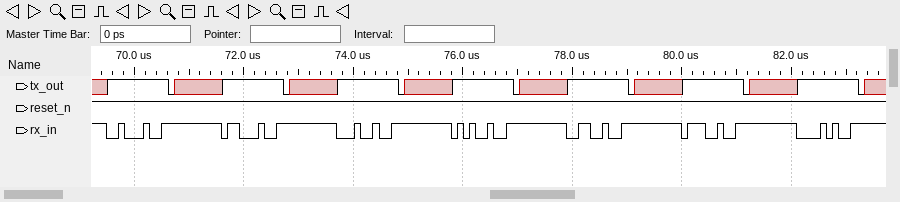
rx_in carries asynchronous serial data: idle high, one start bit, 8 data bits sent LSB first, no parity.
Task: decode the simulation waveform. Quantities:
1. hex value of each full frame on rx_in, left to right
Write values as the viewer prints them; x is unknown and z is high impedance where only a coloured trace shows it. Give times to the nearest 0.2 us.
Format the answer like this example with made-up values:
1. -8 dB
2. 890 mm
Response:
1. 22, 23, 24, 25, 26, 27, 28
